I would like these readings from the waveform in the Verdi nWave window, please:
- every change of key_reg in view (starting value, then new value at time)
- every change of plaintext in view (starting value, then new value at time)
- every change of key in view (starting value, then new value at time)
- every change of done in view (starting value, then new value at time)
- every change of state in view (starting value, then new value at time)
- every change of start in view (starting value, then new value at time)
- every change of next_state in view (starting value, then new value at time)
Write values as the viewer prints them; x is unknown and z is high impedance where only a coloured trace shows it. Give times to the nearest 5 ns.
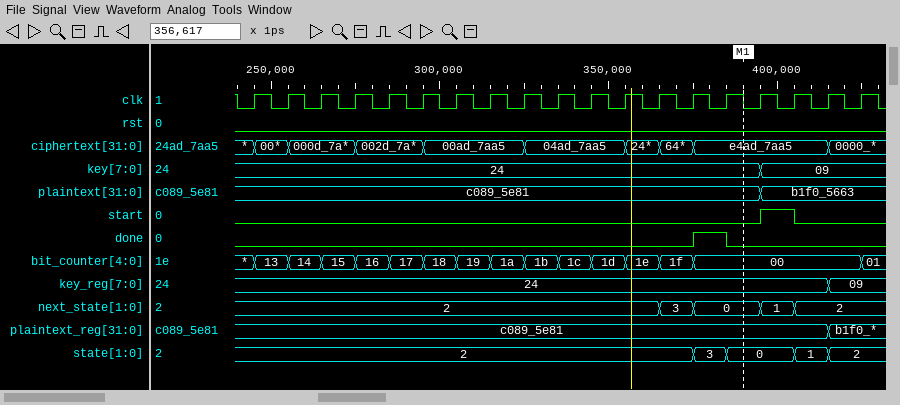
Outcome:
24, 09 at 415 ns
c089_5e81, b1f0_5663 at 395 ns
24, 09 at 395 ns
0, 1 at 375 ns, 0 at 385 ns
2, 3 at 375 ns, 0 at 385 ns, 1 at 405 ns, 2 at 415 ns
0, 1 at 395 ns, 0 at 405 ns
2, 3 at 365 ns, 0 at 375 ns, 1 at 395 ns, 2 at 405 ns
